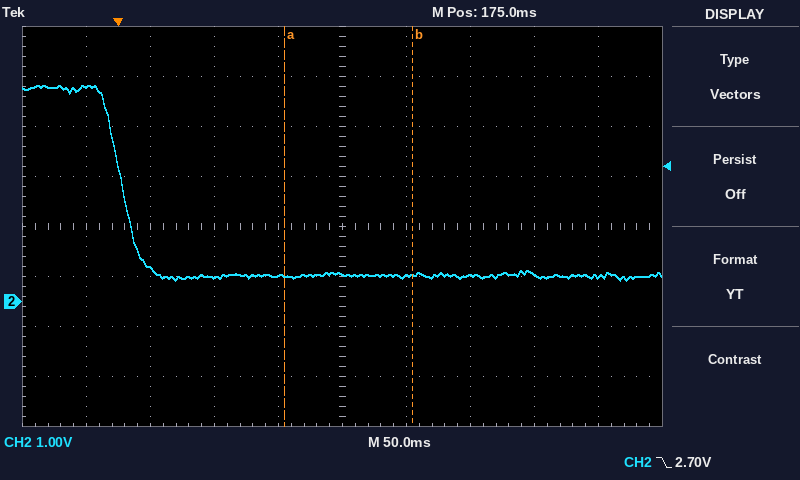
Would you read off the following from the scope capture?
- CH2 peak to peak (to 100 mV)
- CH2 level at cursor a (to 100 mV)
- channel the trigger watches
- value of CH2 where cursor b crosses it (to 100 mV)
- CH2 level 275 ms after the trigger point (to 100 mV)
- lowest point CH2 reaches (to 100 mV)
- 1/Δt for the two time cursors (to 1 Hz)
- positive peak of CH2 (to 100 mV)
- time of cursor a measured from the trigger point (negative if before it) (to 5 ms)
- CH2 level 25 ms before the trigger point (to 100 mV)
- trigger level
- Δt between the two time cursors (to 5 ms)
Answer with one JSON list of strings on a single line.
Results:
["3.9 V", "500 mV", "CH2", "500 mV", "500 mV", "400 mV", "10 Hz", "4.3 V", "+130 ms", "4.3 V", "2.70 V", "100 ms"]
